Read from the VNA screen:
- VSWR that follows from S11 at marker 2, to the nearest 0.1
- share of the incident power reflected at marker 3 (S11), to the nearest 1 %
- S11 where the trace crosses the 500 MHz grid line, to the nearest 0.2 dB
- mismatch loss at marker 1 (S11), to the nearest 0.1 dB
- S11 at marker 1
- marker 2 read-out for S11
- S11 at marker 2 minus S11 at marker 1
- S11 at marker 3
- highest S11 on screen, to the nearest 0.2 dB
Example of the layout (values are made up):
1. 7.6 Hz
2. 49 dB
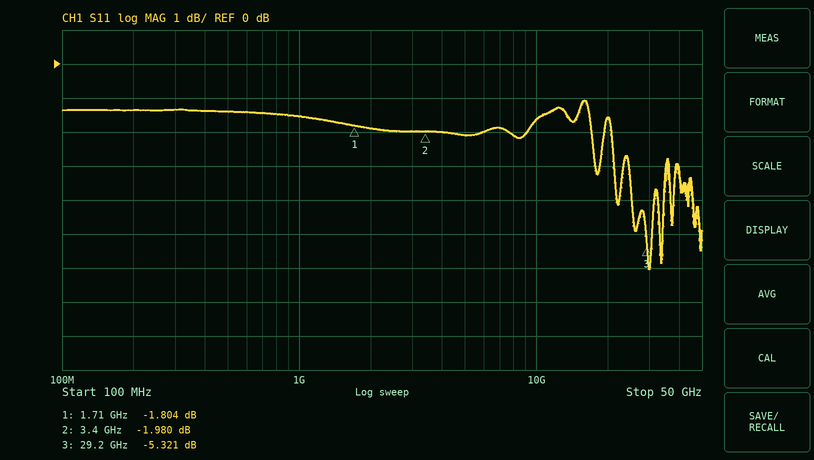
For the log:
1. 8.8
2. 29 %
3. -1.4 dB
4. 4.7 dB
5. -1.804 dB
6. -1.980 dB
7. -0.176 dB
8. -5.321 dB
9. -1.0 dB
